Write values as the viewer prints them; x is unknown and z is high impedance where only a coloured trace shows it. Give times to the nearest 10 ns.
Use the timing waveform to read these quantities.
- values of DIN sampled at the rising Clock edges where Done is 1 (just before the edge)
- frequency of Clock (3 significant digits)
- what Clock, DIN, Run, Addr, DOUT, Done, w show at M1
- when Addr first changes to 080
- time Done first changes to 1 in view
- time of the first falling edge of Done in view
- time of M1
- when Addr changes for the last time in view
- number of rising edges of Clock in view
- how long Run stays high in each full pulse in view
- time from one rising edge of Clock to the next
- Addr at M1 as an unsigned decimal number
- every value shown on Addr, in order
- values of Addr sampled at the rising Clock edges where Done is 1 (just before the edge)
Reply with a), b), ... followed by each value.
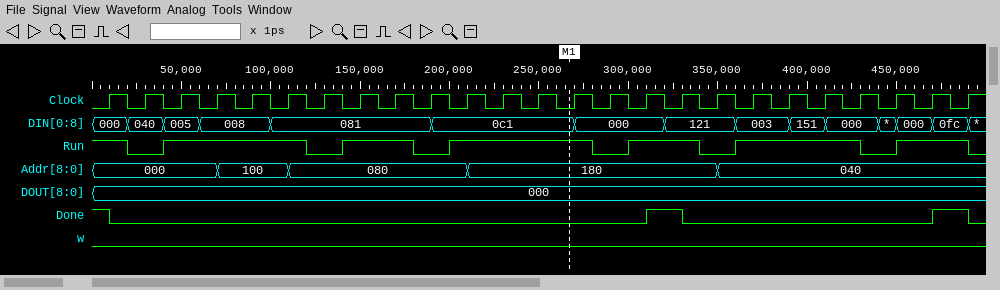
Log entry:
a) 000, 121, 0fc
b) 50.0 MHz
c) Clock=0, DIN=0c1, Run=1, Addr=180, DOUT=000, Done=0, w=0
d) 110 ns
e) 310 ns
f) 10 ns
g) 270 ns
h) 350 ns
i) 25
j) 80 ns, 40 ns, 80 ns, 40 ns, 70 ns, 40 ns
k) 20 ns
l) 384
m) 000, 100, 080, 180, 040
n) 000, 180, 040
